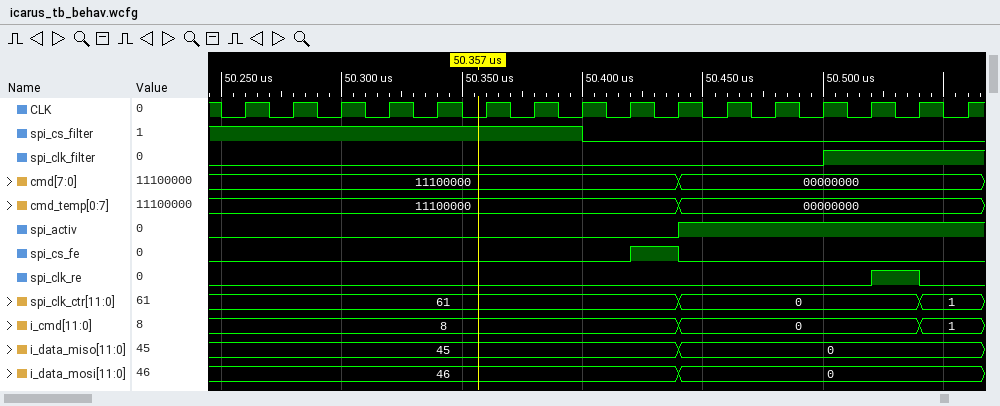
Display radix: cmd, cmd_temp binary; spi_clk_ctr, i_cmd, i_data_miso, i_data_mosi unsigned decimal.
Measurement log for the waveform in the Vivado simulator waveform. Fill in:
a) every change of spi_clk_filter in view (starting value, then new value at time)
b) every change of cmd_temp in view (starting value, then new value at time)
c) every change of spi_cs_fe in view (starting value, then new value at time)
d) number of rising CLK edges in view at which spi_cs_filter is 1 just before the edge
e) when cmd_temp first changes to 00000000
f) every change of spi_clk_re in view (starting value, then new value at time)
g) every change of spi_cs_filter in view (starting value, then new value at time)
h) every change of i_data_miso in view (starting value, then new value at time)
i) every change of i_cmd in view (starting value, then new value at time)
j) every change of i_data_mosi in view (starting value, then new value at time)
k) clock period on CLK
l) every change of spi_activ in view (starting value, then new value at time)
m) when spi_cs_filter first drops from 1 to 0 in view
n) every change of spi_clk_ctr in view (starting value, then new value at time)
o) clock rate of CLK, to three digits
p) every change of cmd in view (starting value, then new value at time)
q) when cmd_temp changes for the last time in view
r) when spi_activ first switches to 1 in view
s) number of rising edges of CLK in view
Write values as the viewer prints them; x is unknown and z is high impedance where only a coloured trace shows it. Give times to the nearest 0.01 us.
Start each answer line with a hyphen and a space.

- 0, 1 at 50.5 us
- 11100000, 00000000 at 50.44 us
- 0, 1 at 50.42 us, 0 at 50.44 us
- 8
- 50.44 us
- 0, 1 at 50.52 us, 0 at 50.54 us
- 1, 0 at 50.4 us
- 45, 0 at 50.44 us
- 8, 0 at 50.44 us, 1 at 50.54 us
- 46, 0 at 50.44 us
- 0.02 us
- 0, 1 at 50.44 us
- 50.4 us
- 61, 0 at 50.44 us, 1 at 50.54 us
- 50.0 MHz
- 11100000, 00000000 at 50.44 us
- 50.44 us
- 50.44 us
- 16
